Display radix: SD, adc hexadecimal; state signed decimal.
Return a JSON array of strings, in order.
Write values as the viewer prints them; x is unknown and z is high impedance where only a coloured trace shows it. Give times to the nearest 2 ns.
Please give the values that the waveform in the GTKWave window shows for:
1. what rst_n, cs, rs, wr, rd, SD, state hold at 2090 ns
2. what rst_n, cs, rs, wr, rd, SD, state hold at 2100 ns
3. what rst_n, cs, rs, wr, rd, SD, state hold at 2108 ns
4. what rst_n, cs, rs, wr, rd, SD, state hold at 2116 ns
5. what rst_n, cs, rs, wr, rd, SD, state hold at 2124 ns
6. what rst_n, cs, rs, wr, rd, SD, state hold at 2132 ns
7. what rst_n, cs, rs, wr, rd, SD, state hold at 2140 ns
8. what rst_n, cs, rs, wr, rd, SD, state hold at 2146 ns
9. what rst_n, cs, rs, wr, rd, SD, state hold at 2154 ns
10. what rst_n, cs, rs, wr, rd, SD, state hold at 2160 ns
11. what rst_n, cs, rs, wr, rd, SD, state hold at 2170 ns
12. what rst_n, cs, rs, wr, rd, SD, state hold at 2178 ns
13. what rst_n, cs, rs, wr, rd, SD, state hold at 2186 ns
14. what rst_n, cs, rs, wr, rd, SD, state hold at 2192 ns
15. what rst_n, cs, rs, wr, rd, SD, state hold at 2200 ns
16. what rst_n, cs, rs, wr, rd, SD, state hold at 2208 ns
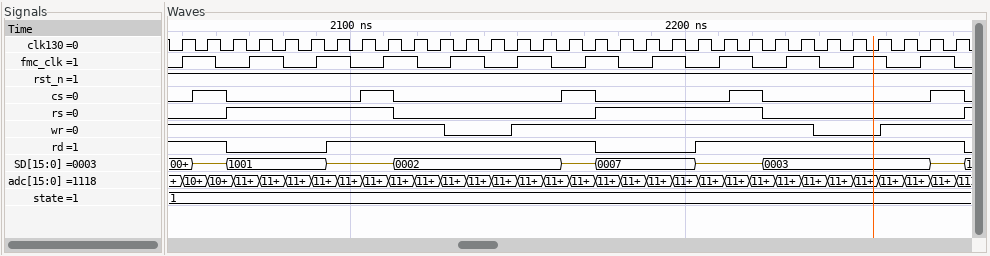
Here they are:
["rst_n=1, cs=0, rs=1, wr=1, rd=0, SD=1001, state=1", "rst_n=1, cs=0, rs=1, wr=1, rd=1, SD=z, state=1", "rst_n=1, cs=1, rs=1, wr=1, rd=1, SD=z, state=1", "rst_n=1, cs=0, rs=0, wr=1, rd=1, SD=0002, state=1", "rst_n=1, cs=0, rs=0, wr=1, rd=1, SD=0002, state=1", "rst_n=1, cs=0, rs=0, wr=0, rd=1, SD=0002, state=1", "rst_n=1, cs=0, rs=0, wr=0, rd=1, SD=0002, state=1", "rst_n=1, cs=0, rs=0, wr=0, rd=1, SD=0002, state=1", "rst_n=1, cs=0, rs=0, wr=1, rd=1, SD=0002, state=1", "rst_n=1, cs=0, rs=0, wr=1, rd=1, SD=0002, state=1", "rst_n=1, cs=1, rs=0, wr=1, rd=1, SD=z, state=1", "rst_n=1, cs=0, rs=1, wr=1, rd=0, SD=0007, state=1", "rst_n=1, cs=0, rs=1, wr=1, rd=0, SD=0007, state=1", "rst_n=1, cs=0, rs=1, wr=1, rd=0, SD=0007, state=1", "rst_n=1, cs=0, rs=1, wr=1, rd=0, SD=0007, state=1", "rst_n=1, cs=0, rs=1, wr=1, rd=1, SD=z, state=1"]
